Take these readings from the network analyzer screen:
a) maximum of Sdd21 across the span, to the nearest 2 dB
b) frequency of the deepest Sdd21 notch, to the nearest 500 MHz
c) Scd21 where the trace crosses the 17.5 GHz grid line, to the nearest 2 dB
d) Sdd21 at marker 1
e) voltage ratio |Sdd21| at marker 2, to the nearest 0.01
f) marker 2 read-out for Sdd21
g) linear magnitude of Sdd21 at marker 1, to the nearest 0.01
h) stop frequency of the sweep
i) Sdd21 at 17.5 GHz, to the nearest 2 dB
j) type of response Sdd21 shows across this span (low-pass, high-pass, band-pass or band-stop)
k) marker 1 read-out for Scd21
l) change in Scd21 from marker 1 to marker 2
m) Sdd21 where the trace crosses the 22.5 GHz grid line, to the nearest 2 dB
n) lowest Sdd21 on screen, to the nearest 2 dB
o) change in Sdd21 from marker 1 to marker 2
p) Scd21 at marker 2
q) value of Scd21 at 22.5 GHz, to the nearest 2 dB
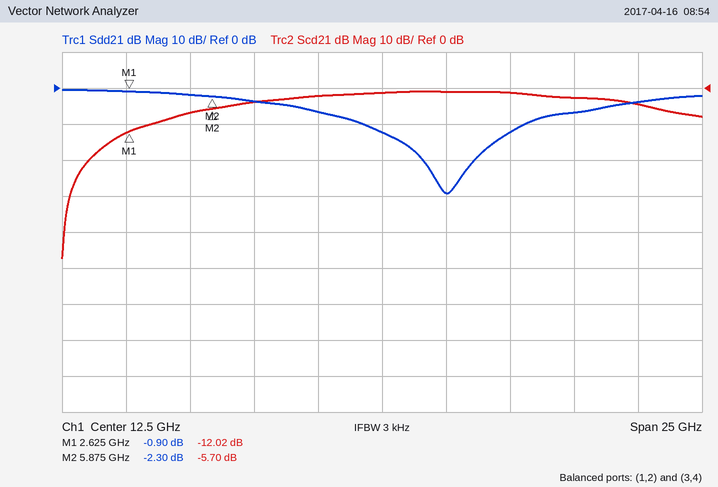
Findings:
0 dB
15.0 GHz
-2 dB
-0.90 dB
0.77
-2.30 dB
0.90
25 GHz
-12 dB
band-stop
-12.02 dB
6.32 dB
-4 dB
-30 dB
-1.40 dB
-5.70 dB
-4 dB
